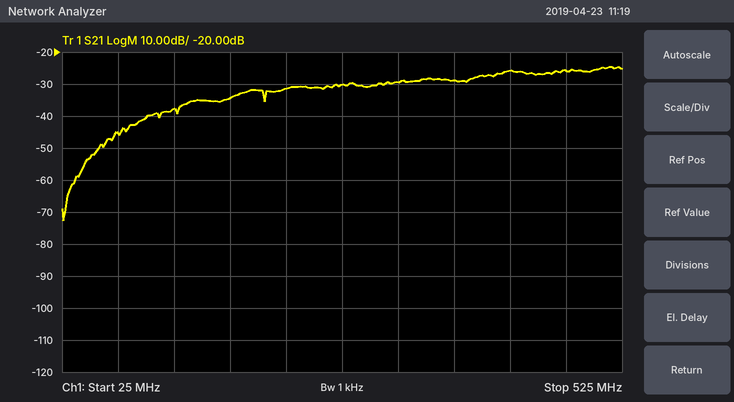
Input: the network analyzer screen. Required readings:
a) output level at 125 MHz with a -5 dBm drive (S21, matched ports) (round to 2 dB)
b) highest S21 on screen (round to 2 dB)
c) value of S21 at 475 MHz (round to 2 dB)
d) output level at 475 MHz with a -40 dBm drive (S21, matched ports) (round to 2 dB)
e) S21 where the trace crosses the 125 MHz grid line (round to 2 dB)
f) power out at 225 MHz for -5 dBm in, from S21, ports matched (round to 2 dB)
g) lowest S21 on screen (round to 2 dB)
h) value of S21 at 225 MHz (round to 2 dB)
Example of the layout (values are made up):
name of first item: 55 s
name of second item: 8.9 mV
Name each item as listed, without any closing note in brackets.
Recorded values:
output level at 125 MHz with a -5 dBm drive (S21, matched ports): -42 dBm
highest S21 on screen: -24 dB
value of S21 at 475 MHz: -26 dB
output level at 475 MHz with a -40 dBm drive (S21, matched ports): -66 dBm
S21 where the trace crosses the 125 MHz grid line: -38 dB
power out at 225 MHz for -5 dBm in, from S21, ports matched: -36 dBm
lowest S21 on screen: -72 dB
value of S21 at 225 MHz: -32 dB
